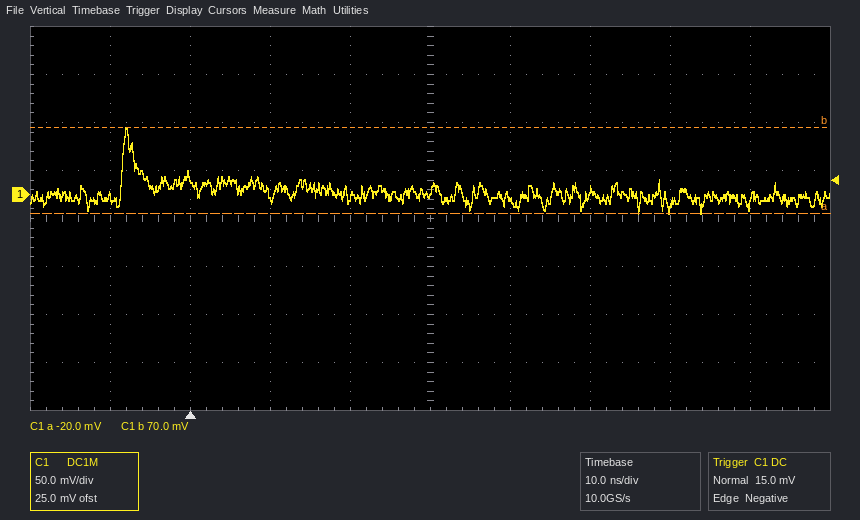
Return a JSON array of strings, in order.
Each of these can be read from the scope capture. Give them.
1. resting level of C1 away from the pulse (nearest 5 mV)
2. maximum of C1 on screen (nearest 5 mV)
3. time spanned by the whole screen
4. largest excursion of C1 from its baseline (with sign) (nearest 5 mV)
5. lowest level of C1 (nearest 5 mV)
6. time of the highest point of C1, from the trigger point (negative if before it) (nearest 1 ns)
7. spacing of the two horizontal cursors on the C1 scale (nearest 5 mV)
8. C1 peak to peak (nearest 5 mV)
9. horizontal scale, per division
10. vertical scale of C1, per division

["0 mV", "70 mV", "100 ns", "+70 mV", "-20 mV", "-8 ns", "90 mV", "90 mV", "10 ns", "50 mV"]
